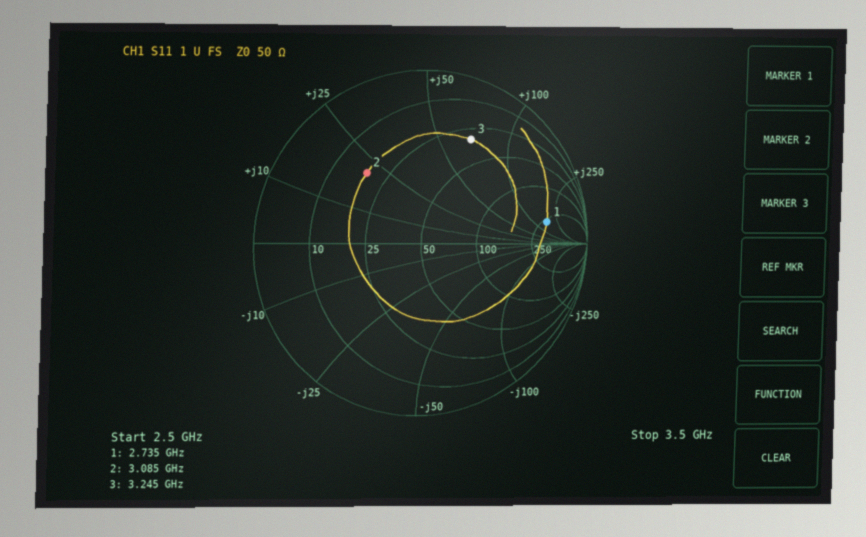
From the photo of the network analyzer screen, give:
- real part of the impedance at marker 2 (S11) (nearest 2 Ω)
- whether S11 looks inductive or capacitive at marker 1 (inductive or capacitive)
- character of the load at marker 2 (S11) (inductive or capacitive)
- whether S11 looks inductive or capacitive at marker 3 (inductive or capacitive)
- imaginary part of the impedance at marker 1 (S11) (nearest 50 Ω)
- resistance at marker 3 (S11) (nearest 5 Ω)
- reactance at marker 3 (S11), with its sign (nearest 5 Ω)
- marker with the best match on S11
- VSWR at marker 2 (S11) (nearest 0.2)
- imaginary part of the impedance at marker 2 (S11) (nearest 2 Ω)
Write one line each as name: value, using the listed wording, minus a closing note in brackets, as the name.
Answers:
real part of the impedance at marker 2 (S11): 18 Ω
whether S11 looks inductive or capacitive at marker 1: inductive
character of the load at marker 2 (S11): inductive
whether S11 looks inductive or capacitive at marker 3: inductive
imaginary part of the impedance at marker 1 (S11): +150 Ω
resistance at marker 3 (S11): 30 Ω
reactance at marker 3 (S11), with its sign: +70 Ω
marker with the best match on S11: marker 2
VSWR at marker 2 (S11): 3.2
imaginary part of the impedance at marker 2 (S11): +20 Ω
